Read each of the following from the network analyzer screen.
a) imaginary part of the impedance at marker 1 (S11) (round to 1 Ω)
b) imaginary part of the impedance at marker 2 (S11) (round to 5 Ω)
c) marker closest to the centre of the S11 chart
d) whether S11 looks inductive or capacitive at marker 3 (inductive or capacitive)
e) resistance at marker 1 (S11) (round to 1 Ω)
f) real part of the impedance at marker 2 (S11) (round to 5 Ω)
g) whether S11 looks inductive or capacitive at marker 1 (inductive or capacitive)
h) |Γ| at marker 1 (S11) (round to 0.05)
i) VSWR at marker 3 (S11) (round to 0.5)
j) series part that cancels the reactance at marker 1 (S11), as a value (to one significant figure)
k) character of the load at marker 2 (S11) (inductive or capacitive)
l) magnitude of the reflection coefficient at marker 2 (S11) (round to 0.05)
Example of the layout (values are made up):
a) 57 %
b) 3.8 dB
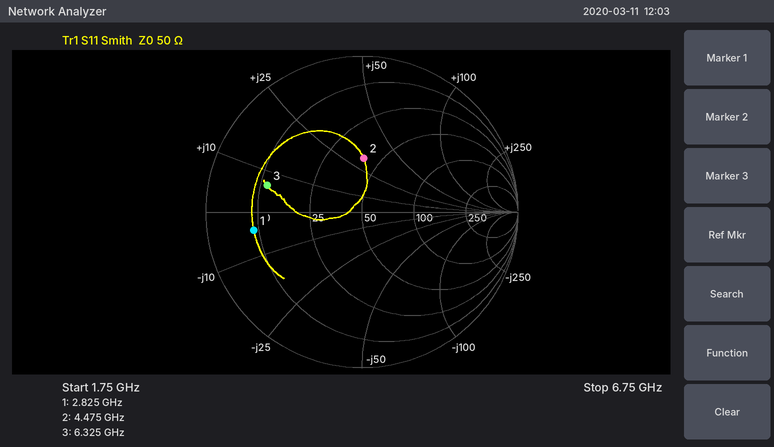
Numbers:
a) -4 Ω
b) +30 Ω
c) marker 2
d) inductive
e) 9 Ω
f) 40 Ω
g) capacitive
h) 0.70
i) 4.5
j) 200 pH
k) inductive
l) 0.35
